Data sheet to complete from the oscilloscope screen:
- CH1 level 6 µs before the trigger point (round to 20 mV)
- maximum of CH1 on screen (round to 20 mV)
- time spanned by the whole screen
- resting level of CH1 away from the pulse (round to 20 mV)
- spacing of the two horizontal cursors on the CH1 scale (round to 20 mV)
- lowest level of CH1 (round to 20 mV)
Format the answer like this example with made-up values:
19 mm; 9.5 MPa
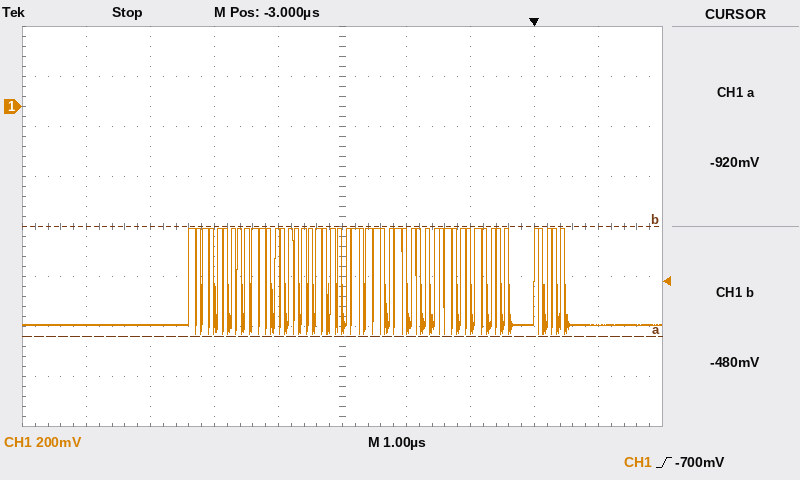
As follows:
-880 mV; -480 mV; 10 µs; -880 mV; 440 mV; -920 mV
